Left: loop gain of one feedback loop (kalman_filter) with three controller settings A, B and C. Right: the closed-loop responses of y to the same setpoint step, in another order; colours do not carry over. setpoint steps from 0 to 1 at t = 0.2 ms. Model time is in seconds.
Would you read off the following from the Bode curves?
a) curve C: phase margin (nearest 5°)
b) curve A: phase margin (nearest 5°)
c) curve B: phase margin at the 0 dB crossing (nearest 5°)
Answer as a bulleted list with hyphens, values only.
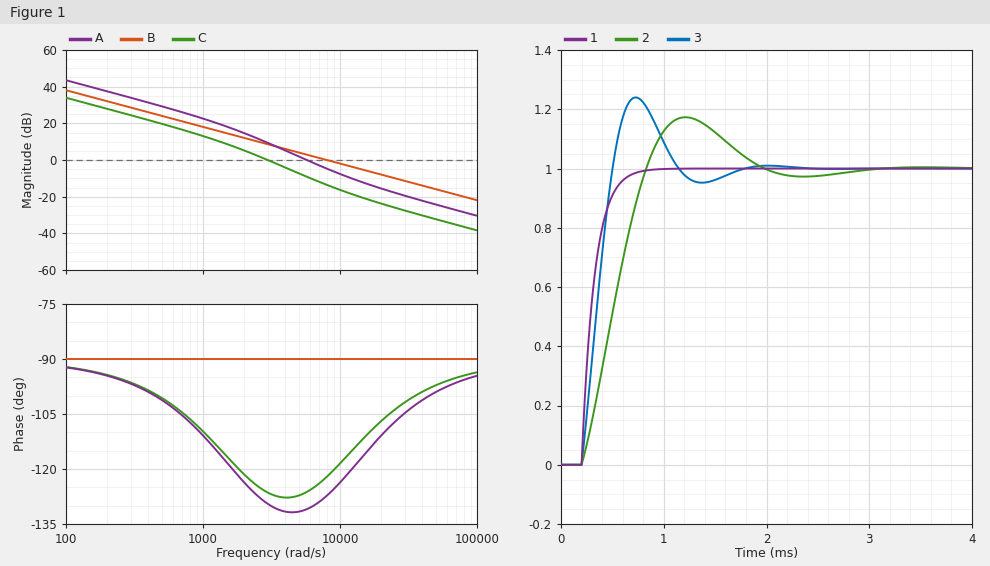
- 55°
- 50°
- 90°
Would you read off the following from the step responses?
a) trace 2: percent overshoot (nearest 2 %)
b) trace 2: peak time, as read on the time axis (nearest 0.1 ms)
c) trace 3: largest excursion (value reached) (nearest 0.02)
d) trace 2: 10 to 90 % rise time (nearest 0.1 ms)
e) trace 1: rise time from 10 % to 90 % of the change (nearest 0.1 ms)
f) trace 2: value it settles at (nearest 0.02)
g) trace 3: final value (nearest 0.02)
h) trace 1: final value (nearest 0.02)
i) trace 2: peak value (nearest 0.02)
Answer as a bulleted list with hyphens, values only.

- 18 %
- 1.2 ms
- 1.24
- 0.5 ms
- 0.3 ms
- 1.00
- 1.00
- 1.00
- 1.18
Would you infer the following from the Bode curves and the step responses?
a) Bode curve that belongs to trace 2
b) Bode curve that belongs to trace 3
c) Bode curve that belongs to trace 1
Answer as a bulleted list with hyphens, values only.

- C
- A
- B
